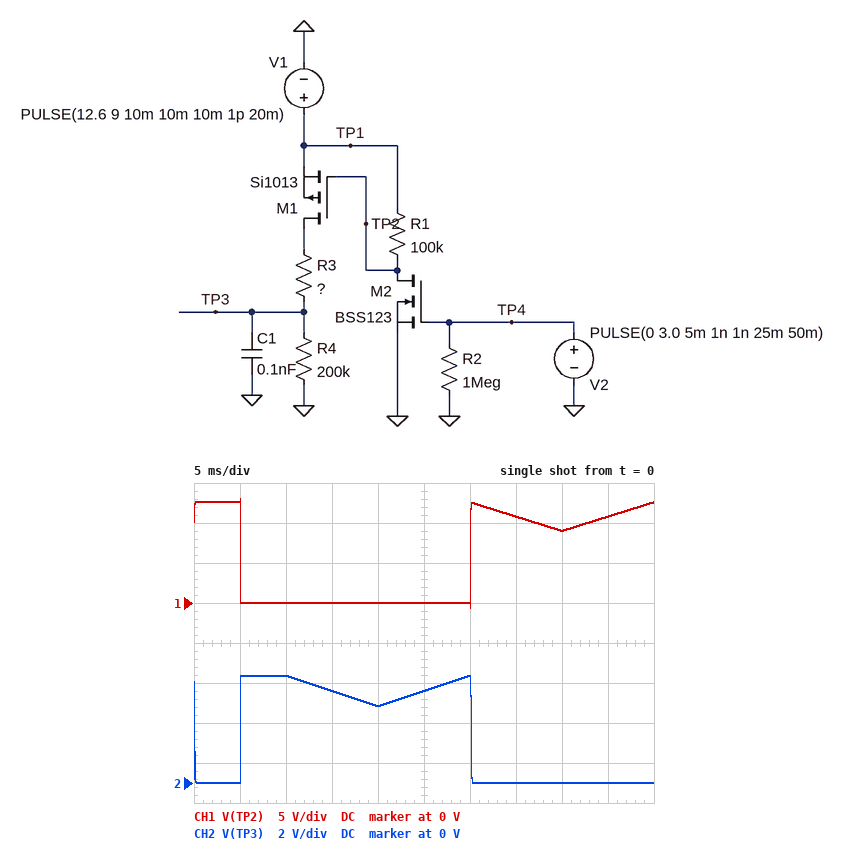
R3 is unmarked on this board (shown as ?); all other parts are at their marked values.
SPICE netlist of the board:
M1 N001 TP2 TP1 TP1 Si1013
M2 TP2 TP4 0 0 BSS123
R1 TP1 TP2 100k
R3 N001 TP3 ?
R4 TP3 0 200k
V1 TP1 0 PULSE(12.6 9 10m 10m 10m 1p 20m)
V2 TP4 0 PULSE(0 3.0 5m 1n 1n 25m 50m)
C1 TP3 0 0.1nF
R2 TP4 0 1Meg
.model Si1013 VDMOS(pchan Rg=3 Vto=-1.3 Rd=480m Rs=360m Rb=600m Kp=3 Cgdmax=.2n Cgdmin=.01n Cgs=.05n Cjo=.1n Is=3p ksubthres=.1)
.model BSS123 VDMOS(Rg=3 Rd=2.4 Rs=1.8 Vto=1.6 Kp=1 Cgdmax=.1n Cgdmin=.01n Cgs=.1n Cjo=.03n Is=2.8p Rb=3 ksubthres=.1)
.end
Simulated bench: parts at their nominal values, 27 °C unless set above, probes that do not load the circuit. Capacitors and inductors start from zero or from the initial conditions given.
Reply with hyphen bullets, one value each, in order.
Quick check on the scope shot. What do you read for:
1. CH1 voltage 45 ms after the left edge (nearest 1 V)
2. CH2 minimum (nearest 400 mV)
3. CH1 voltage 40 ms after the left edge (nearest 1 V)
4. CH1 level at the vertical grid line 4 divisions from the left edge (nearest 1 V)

- 11 V
- 0 V
- 9 V
- 0 V
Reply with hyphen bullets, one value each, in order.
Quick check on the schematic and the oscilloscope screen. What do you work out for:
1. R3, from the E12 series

- 270 kΩ
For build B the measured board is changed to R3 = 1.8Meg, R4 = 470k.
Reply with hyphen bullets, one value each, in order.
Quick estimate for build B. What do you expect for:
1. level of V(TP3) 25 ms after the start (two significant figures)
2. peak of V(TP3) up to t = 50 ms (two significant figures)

- 2.2 V
- 2.6 V
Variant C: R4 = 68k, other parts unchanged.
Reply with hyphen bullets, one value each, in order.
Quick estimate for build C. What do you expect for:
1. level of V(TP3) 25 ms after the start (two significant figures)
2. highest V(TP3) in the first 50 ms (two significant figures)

- 2.2 V
- 2.5 V
